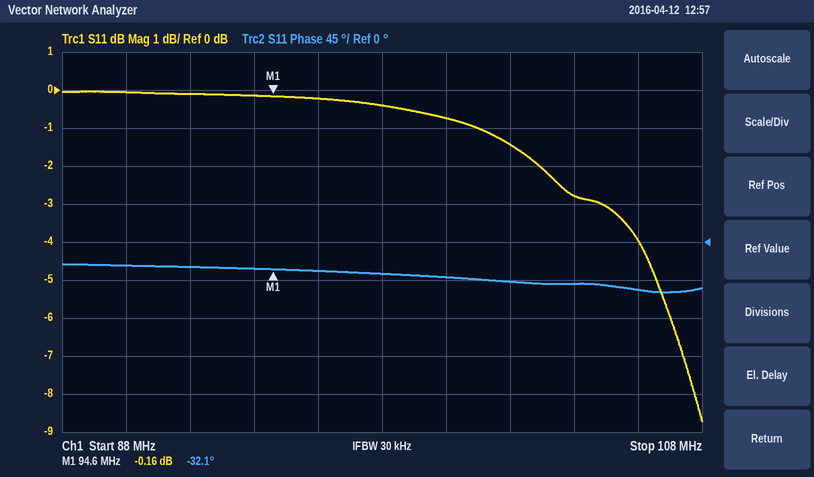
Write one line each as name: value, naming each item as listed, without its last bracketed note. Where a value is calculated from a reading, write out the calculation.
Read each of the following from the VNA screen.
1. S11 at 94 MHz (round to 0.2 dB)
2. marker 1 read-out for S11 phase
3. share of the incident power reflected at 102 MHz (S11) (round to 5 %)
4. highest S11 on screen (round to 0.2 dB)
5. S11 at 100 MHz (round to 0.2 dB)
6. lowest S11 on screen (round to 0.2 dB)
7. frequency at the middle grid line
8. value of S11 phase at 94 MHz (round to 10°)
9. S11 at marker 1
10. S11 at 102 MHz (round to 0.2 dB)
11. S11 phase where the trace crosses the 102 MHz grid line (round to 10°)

S11 at 94 MHz: -0.2 dB
marker 1 read-out for S11 phase: -32.1°
share of the incident power reflected at 102 MHz (S11): 10^(-1.4/10) ≈ 72.4 %, so 70 % to the nearest 5 %
highest S11 on screen: 0.0 dB
S11 at 100 MHz: -0.8 dB
lowest S11 on screen: -8.8 dB
frequency at the middle grid line: 98 MHz
value of S11 phase at 94 MHz: -30°
S11 at marker 1: -0.16 dB
S11 at 102 MHz: -1.4 dB
S11 phase where the trace crosses the 102 MHz grid line: -50°
